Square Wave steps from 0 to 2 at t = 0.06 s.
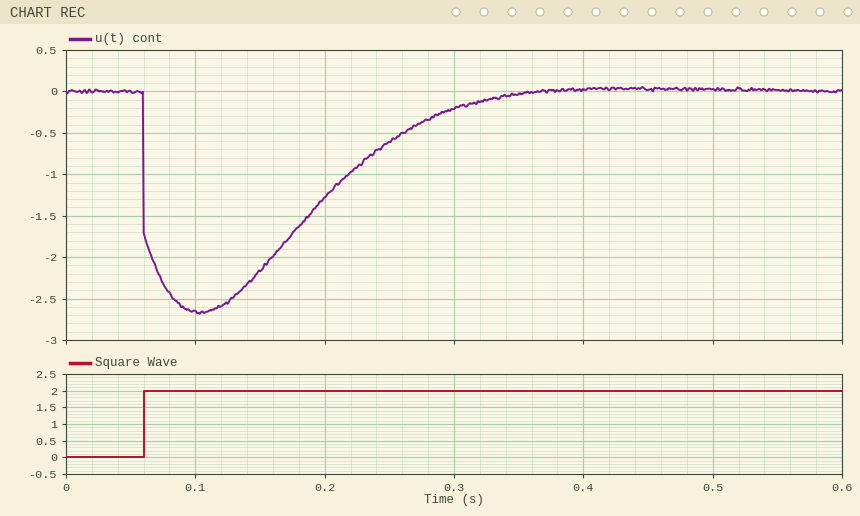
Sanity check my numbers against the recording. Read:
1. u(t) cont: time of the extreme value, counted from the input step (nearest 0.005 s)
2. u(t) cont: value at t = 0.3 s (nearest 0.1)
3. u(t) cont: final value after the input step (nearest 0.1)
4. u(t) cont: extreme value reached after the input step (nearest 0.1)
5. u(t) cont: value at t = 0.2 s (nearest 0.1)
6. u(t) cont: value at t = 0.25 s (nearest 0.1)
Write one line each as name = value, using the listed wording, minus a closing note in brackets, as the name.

u(t) cont: time of the extreme value, counted from the input step = 0.045 s
u(t) cont: value at t = 0.3 s = -0.2
u(t) cont: final value after the input step = 0.0
u(t) cont: extreme value reached after the input step = -2.7
u(t) cont: value at t = 0.2 s = -1.3
u(t) cont: value at t = 0.25 s = -0.6
